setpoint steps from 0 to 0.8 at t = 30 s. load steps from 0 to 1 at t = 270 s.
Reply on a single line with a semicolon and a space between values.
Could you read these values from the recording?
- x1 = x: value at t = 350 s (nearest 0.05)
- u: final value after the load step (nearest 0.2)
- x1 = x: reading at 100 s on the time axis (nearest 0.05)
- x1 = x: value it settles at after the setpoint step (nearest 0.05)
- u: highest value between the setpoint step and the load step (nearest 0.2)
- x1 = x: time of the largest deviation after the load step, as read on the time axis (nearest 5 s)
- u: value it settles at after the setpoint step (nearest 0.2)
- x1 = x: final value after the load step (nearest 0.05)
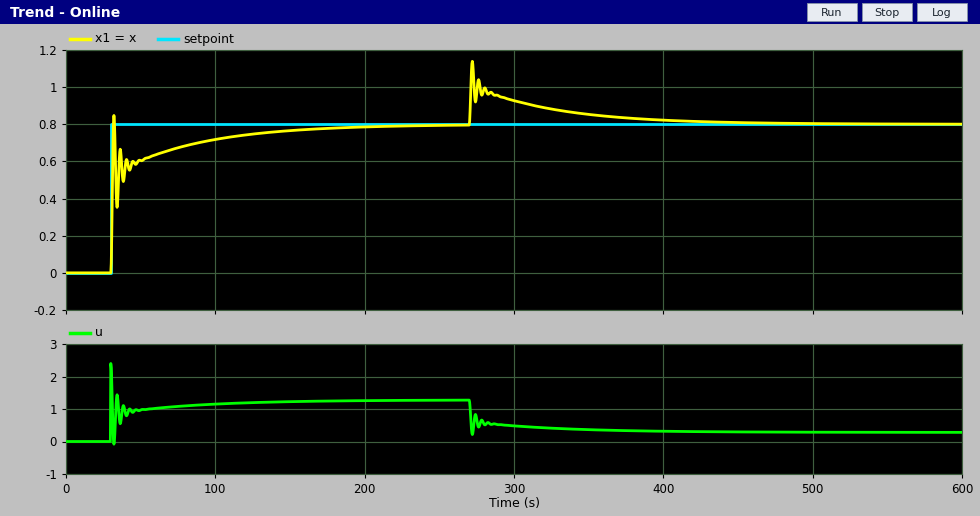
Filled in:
0.85; 0.2; 0.70; 0.80; 2.4; 270 s; 1.2; 0.80
